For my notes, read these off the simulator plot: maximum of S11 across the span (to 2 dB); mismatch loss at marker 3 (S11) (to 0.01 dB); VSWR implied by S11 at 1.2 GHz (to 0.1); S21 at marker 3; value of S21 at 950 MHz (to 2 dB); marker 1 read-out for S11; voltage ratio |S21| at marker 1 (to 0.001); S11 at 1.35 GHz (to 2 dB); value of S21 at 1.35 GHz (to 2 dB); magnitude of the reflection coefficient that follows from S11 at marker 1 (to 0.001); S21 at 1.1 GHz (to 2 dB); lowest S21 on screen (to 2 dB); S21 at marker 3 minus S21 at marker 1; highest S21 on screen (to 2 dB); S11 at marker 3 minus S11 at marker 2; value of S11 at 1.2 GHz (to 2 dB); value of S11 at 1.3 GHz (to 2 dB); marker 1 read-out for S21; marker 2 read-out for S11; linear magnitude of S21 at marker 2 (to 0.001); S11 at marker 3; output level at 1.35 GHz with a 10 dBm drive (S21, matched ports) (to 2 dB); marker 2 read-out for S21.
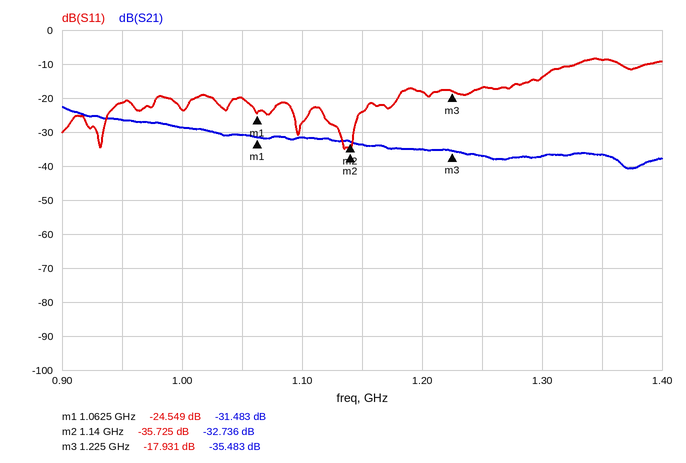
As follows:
-8 dB
0.07 dB
1.3
-35.483 dB
-26 dB
-24.549 dB
0.027
-8 dB
-36 dB
0.059
-32 dB
-40 dB
-4.000 dB
-22 dB
17.794 dB
-18 dB
-14 dB
-31.483 dB
-35.725 dB
0.023
-17.931 dB
-26 dBm
-32.736 dB
